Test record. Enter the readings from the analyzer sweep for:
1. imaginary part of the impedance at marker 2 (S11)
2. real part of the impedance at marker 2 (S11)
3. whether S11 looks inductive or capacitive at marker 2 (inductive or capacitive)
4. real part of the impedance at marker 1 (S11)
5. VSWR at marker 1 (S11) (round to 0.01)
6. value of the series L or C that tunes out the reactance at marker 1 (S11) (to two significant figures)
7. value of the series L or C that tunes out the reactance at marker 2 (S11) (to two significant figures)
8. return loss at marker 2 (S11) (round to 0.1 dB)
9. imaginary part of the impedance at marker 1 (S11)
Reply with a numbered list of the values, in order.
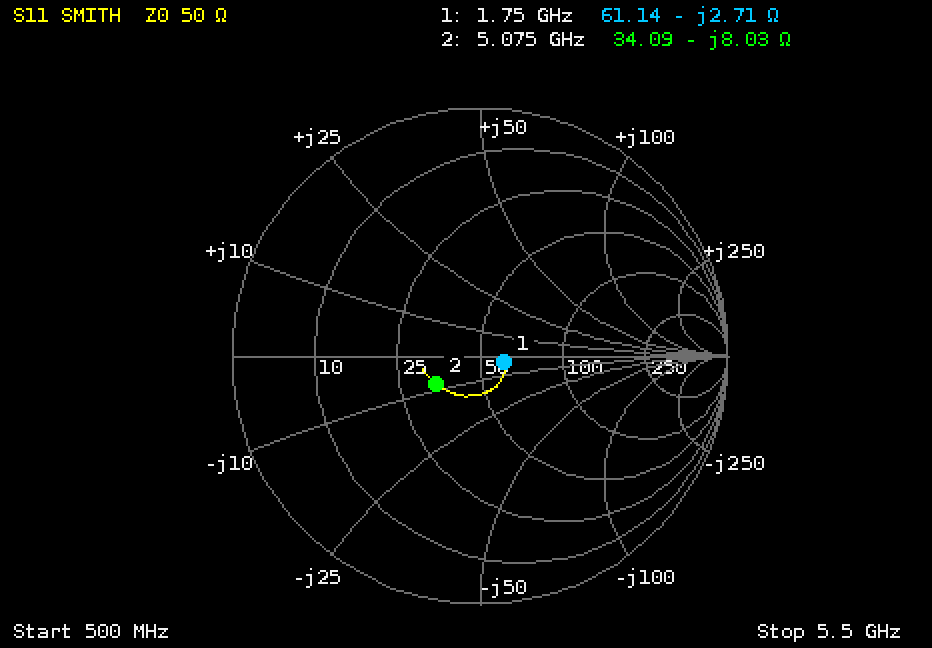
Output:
1. -8.03 Ω
2. 34.09 Ω
3. capacitive
4. 61.14 Ω
5. 1.23
6. 250 pH
7. 250 pH
8. 13.5 dB
9. -2.71 Ω
